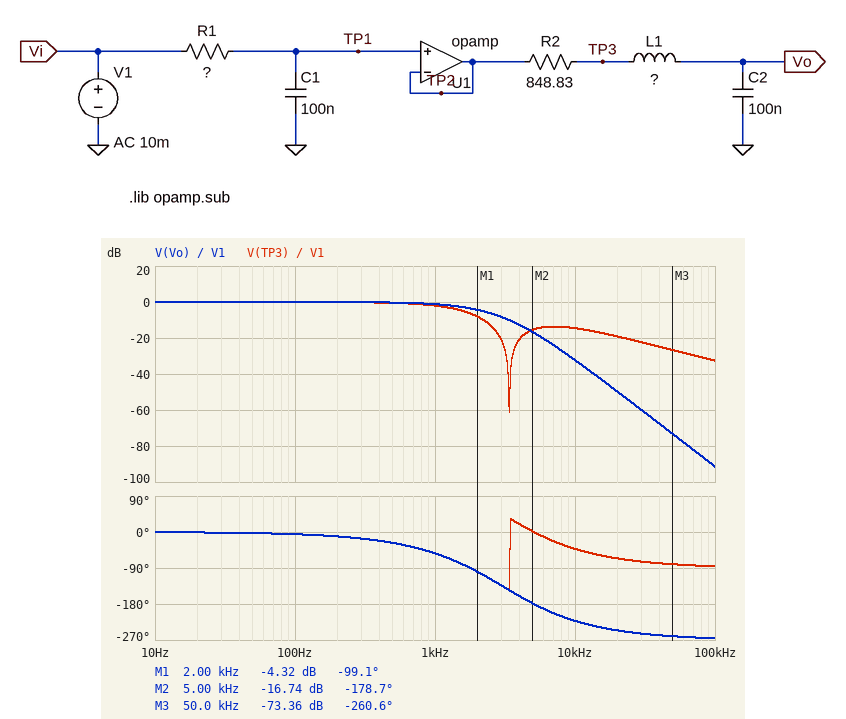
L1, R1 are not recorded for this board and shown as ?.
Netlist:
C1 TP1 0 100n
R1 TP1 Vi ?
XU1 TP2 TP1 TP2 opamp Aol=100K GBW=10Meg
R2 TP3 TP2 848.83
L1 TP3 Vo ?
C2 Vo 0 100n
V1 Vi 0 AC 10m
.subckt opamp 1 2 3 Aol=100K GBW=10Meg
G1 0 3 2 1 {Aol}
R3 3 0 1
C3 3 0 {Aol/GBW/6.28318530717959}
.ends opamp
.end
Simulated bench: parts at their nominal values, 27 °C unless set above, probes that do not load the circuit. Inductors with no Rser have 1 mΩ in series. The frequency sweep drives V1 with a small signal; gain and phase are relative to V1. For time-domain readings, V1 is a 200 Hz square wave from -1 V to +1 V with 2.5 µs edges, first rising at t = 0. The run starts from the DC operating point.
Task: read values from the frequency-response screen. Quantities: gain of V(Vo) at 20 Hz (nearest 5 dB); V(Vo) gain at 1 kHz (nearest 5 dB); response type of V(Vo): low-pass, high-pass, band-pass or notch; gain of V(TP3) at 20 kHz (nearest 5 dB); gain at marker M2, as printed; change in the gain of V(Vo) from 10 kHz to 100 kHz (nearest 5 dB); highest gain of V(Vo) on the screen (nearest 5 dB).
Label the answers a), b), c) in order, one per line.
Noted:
a) 0 dB
b) 0 dB
c) low-pass
d) -20 dB
e) -16.74 dB
f) -60 dB
g) 0 dB
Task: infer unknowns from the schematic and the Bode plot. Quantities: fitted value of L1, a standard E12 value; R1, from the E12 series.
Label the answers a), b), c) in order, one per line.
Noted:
a) 22 mH
b) 680 Ω
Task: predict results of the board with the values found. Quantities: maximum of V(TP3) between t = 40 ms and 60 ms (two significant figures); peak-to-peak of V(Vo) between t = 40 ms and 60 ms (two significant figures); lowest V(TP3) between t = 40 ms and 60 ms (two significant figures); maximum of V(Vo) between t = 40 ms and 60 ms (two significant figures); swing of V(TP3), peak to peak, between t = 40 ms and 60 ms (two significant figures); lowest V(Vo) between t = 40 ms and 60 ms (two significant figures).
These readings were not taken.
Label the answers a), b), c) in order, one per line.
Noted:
a) 1.0 V
b) 2.0 V
c) -1.0 V
d) 1.0 V
e) 2.0 V
f) -1.0 V
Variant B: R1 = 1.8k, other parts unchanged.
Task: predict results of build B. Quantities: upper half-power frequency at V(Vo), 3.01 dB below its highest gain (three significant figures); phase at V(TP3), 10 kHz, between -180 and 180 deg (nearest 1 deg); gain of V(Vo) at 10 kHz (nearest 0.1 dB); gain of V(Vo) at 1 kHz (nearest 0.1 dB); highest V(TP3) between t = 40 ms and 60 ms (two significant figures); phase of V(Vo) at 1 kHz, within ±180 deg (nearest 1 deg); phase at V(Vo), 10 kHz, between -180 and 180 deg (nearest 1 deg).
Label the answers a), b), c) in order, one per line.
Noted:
a) 818 Hz
b) -50 deg
c) -40.5 dB
d) -4.1 dB
e) 1.0 V
f) -79 deg
g) 130 deg
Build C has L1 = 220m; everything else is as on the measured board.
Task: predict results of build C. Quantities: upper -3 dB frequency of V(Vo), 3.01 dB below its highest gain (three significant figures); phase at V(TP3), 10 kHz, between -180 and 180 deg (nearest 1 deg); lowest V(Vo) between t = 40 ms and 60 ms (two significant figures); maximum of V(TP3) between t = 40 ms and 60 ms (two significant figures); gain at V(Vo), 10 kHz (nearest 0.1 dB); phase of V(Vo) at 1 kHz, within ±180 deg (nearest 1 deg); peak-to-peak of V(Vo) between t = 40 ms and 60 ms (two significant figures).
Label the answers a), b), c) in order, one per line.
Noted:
a) 1.24 kHz
b) -73 deg
c) -1.7 V
d) 1.3 V
e) -51.5 dB
f) -99 deg
g) 3.4 V
